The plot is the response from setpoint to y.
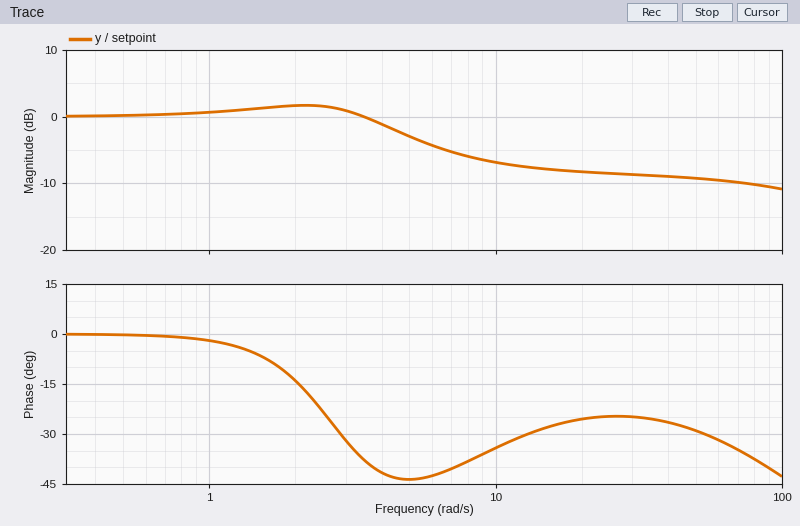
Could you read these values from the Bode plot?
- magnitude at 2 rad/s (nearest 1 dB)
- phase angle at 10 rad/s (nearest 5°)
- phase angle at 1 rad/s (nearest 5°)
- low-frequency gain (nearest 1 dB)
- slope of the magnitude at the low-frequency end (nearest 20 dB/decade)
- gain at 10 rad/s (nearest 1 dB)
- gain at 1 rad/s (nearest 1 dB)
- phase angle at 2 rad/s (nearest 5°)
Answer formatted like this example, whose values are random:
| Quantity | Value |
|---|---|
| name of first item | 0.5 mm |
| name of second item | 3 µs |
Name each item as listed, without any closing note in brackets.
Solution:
| Quantity | Value |
|---|---|
| magnitude at 2 rad/s | 2 dB |
| phase angle at 10 rad/s | -35° |
| phase angle at 1 rad/s | 0° |
| low-frequency gain | 0 dB |
| slope of the magnitude at the low-frequency end | 0 dB/decade |
| gain at 10 rad/s | -7 dB |
| gain at 1 rad/s | 1 dB |
| phase angle at 2 rad/s | -15° |
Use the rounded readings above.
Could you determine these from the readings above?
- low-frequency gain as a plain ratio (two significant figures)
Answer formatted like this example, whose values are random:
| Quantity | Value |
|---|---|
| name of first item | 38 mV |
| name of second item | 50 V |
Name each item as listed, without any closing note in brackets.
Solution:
| Quantity | Value |
|---|---|
| low-frequency gain as a plain ratio | 1.0 |
